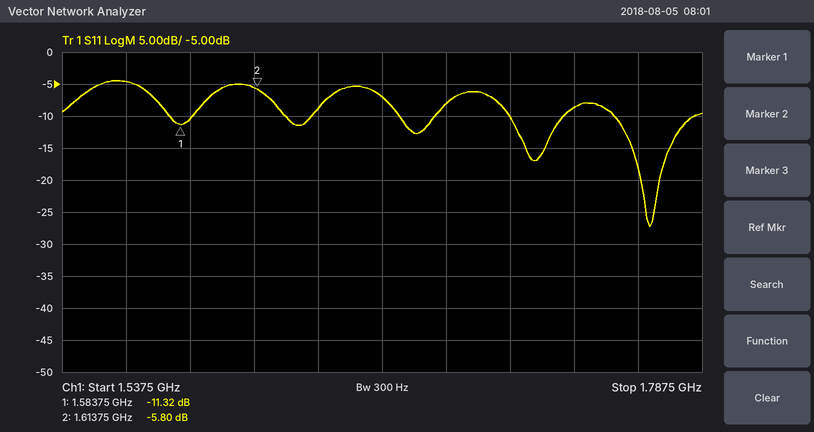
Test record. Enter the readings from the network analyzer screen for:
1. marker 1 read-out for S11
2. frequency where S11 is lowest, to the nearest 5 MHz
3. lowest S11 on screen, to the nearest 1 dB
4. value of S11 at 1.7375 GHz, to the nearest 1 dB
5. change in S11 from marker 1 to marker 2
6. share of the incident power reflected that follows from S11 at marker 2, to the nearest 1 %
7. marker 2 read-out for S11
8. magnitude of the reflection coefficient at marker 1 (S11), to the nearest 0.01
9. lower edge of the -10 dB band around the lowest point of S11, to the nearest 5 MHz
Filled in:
-11.32 dB
1.765 GHz
-27 dB
-9 dB
5.52 dB
26 %
-5.80 dB
0.27
1.755 GHz
